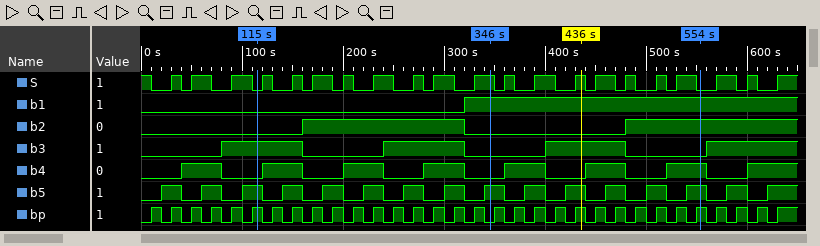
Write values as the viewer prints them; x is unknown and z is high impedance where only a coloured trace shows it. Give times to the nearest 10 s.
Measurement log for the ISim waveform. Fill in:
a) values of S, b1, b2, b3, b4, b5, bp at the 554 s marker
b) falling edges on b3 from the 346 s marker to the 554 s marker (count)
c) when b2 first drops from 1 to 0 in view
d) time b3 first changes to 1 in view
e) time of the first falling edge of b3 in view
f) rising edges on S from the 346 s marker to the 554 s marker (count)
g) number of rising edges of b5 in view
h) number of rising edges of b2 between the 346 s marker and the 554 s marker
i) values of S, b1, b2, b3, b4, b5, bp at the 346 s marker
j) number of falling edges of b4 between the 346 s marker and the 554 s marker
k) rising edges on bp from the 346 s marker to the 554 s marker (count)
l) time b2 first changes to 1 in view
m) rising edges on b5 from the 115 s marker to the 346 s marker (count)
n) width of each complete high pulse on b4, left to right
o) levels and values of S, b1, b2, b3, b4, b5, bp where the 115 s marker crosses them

S=0, b1=1, b2=1, b3=0, b4=1, b5=1, bp=1
1
320 s
80 s
160 s
7
16
1
S=1, b1=1, b2=0, b3=0, b4=0, b5=1, bp=0
2
11
160 s
6
40 s, 40 s, 40 s, 40 s, 40 s, 40 s, 40 s
S=0, b1=0, b2=0, b3=1, b4=0, b5=1, bp=1
